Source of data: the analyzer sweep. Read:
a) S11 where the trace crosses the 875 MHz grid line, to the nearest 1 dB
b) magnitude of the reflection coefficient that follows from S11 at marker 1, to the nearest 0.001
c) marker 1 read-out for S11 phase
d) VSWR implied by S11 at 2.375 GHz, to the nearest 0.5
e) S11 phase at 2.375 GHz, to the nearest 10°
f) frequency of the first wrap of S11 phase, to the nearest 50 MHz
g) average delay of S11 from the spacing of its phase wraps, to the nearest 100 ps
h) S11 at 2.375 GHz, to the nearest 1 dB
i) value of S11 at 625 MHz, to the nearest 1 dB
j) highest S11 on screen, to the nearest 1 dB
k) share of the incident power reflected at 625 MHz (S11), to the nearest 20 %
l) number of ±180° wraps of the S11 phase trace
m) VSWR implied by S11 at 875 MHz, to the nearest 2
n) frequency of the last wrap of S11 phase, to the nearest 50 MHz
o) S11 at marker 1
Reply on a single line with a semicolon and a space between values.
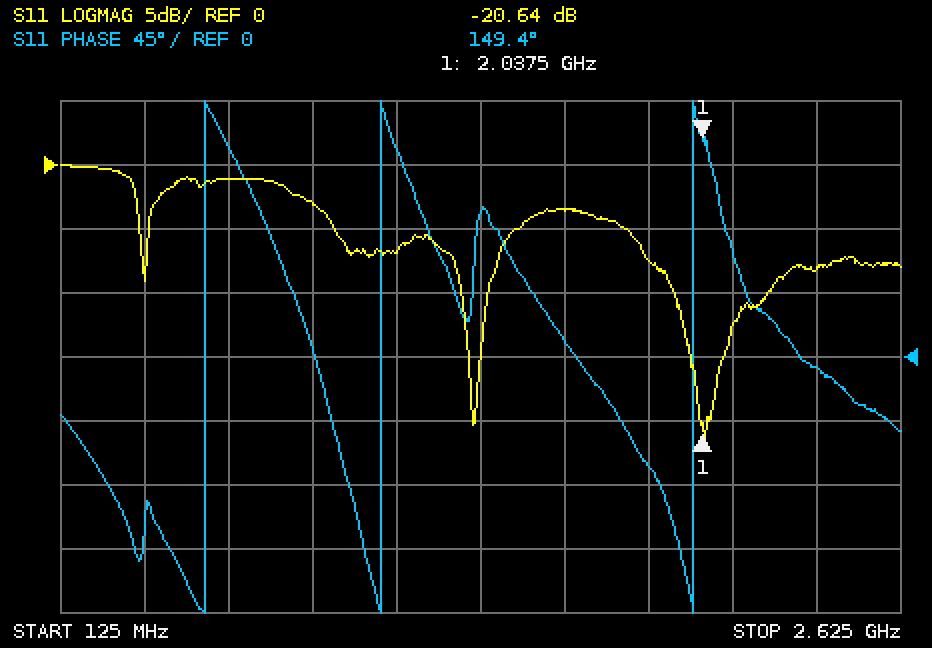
-3 dB; 0.093; 149.4°; 2.5; -10°; 550 MHz; 1.4 ns; -8 dB; -1 dB; 0 dB; 80 %; 3; 6; 2.00 GHz; -20.64 dB
